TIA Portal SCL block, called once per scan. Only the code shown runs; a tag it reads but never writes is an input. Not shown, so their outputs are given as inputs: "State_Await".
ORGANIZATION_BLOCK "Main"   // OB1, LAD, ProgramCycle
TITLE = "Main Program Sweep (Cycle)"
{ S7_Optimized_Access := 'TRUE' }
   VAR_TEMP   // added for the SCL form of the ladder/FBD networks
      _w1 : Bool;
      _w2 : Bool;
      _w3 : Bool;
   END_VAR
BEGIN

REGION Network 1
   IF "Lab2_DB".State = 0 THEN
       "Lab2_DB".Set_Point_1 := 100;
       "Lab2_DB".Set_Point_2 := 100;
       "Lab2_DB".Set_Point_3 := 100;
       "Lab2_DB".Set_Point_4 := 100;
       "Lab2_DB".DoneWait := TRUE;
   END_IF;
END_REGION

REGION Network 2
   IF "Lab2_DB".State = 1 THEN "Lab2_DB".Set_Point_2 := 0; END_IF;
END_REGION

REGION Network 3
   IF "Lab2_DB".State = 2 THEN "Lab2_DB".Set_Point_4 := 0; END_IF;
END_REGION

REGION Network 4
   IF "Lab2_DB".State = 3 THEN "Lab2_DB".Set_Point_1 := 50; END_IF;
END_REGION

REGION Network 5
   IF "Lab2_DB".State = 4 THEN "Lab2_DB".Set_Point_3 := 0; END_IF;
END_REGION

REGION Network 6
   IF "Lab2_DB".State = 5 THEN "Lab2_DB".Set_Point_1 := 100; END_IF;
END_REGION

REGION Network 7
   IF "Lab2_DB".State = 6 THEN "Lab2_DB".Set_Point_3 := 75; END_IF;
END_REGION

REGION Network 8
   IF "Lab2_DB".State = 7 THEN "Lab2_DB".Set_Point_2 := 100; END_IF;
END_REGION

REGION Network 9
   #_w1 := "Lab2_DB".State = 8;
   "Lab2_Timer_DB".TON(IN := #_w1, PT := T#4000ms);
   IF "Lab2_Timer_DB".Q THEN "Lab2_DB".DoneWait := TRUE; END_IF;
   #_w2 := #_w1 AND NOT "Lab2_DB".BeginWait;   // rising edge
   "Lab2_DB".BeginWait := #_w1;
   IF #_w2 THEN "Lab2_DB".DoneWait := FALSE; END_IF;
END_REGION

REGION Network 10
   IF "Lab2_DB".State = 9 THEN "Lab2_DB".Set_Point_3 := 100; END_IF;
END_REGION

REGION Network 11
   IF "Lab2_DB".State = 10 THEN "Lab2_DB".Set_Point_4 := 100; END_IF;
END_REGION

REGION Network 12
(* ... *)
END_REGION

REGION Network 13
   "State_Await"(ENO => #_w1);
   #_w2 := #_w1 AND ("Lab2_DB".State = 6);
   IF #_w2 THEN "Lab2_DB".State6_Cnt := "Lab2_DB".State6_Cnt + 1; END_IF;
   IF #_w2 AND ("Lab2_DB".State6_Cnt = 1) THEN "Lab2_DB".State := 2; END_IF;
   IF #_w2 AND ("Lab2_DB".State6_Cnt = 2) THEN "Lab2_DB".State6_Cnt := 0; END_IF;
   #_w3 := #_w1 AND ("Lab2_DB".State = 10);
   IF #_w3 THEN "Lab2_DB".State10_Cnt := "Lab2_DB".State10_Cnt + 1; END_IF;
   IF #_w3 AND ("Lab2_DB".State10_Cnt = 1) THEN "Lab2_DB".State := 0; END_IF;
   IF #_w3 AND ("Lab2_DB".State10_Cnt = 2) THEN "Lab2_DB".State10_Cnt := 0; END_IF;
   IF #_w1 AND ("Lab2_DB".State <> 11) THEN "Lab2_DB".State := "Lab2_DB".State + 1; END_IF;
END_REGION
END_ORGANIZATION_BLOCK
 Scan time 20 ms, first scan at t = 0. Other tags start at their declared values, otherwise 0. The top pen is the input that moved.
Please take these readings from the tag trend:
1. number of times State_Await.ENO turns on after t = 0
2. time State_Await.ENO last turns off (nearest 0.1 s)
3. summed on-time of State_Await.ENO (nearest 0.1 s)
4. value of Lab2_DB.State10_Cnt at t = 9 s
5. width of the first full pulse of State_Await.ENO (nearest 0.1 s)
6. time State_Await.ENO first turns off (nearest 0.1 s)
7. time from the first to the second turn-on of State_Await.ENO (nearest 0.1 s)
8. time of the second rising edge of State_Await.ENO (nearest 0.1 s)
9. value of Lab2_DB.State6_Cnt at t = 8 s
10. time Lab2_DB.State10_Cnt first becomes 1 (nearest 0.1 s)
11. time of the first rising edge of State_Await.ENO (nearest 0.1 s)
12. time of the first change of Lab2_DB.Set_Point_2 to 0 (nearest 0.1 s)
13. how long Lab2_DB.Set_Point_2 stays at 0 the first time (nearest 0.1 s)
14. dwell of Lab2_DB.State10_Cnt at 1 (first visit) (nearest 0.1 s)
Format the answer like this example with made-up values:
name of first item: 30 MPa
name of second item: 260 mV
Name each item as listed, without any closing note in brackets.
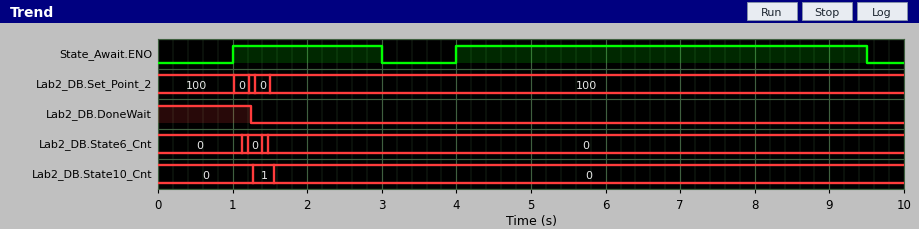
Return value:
number of times State_Await.ENO turns on after t = 0: 2
time State_Await.ENO last turns off: 9.5 s
summed on-time of State_Await.ENO: 7.5 s
value of Lab2_DB.State10_Cnt at t = 9 s: 0
width of the first full pulse of State_Await.ENO: 2.0 s
time State_Await.ENO first turns off: 3.0 s
time from the first to the second turn-on of State_Await.ENO: 3.0 s
time of the second rising edge of State_Await.ENO: 4.0 s
value of Lab2_DB.State6_Cnt at t = 8 s: 0
time Lab2_DB.State10_Cnt first becomes 1: 1.3 s
time of the first rising edge of State_Await.ENO: 1.0 s
time of the first change of Lab2_DB.Set_Point_2 to 0: 1.0 s
how long Lab2_DB.Set_Point_2 stays at 0 the first time: 0.2 s
dwell of Lab2_DB.State10_Cnt at 1 (first visit): 0.3 s
